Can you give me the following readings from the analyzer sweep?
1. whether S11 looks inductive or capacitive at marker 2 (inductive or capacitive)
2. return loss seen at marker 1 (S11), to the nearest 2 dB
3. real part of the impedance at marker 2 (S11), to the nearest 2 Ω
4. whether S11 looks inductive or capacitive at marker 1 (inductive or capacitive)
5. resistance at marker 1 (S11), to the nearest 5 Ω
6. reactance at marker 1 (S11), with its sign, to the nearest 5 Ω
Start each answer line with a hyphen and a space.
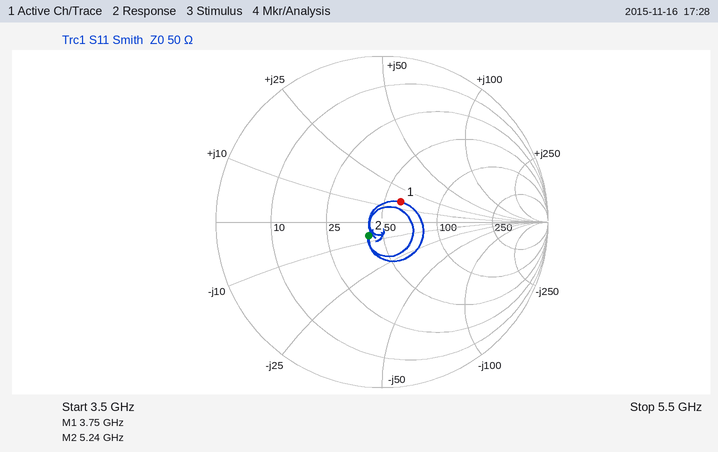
- capacitive
- 16 dB
- 42 Ω
- inductive
- 60 Ω
- +15 Ω
